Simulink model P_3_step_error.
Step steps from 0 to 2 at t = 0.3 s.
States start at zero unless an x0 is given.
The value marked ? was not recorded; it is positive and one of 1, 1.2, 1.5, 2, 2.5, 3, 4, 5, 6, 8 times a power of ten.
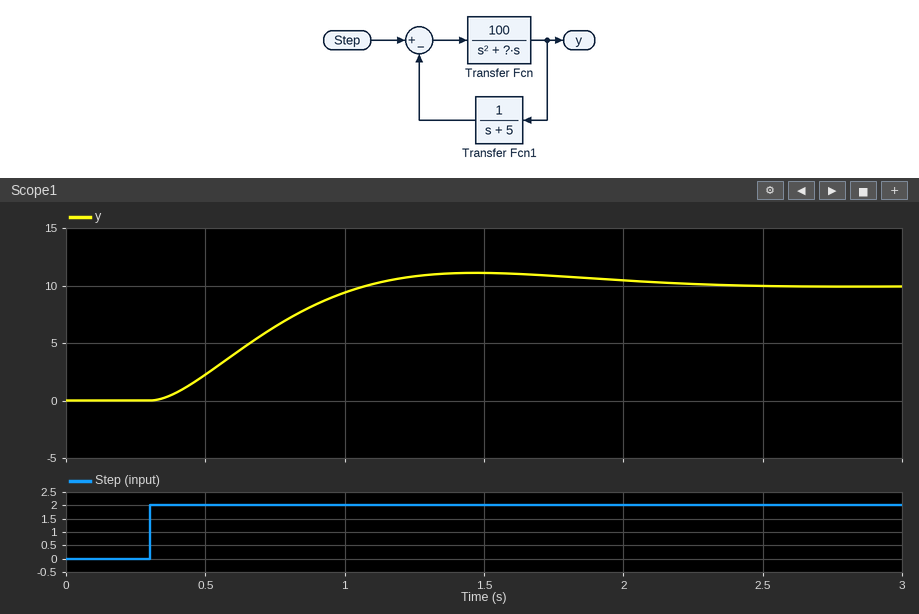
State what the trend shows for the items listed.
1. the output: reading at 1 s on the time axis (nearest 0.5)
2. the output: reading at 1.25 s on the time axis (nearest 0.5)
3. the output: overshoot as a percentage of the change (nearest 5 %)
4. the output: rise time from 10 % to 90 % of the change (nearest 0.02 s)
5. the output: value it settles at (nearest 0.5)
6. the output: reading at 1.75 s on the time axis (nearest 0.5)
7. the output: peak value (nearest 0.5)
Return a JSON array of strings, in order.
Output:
["9.5", "11.0", "10 %", "0.54 s", "10.0", "11.0", "11.0"]
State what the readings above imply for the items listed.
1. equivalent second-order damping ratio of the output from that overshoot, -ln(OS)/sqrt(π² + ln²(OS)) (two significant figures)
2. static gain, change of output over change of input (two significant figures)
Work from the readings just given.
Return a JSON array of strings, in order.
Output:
["0.59", "5.0"]
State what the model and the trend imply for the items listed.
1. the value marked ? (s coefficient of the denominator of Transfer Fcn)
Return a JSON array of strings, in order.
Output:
["10"]
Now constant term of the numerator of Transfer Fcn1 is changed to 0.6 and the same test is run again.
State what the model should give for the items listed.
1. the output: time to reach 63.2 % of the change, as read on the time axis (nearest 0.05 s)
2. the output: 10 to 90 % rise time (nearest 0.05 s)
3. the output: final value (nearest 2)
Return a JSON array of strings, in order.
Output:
["1.00 s", "1.10 s", "16"]
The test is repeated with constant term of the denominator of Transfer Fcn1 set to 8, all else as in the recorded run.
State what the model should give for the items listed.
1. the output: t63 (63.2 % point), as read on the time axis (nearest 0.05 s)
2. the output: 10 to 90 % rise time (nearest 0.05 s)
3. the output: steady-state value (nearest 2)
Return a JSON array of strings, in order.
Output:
["1.00 s", "1.20 s", "16"]
